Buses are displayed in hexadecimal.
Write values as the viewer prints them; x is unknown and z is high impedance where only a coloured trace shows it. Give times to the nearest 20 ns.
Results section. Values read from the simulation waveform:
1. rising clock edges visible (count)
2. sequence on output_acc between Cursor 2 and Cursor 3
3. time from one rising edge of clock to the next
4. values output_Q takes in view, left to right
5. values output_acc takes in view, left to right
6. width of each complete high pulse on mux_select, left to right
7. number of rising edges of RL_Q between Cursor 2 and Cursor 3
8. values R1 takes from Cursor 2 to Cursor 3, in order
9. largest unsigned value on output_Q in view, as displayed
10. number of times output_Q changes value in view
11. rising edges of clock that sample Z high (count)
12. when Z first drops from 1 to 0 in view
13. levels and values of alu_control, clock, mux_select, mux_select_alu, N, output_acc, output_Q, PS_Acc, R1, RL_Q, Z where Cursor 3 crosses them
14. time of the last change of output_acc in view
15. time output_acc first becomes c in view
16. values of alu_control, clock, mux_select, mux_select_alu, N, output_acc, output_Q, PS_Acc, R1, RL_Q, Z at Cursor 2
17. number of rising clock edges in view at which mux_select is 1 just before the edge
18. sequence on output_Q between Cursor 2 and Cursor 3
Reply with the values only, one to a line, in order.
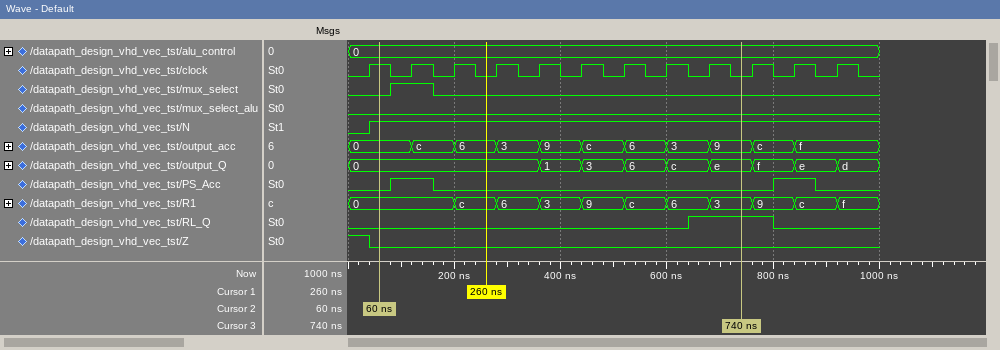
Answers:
12
0, c, 6, 3, 9, c, 6, 3, 9
80 ns
0, 1, 3, 6, c, e, f, e, d
0, c, 6, 3, 9, c, 6, 3, 9, c, f
80 ns
1
0, c, 6, 3, 9, c, 6, 3
f
8
1
40 ns
alu_control=0, clock=0, mux_select=0, mux_select_alu=0, N=1, output_acc=9, output_Q=e, PS_Acc=0, R1=3, RL_Q=1, Z=0
840 ns
120 ns
alu_control=0, clock=1, mux_select=0, mux_select_alu=0, N=1, output_acc=0, output_Q=0, PS_Acc=0, R1=0, RL_Q=0, Z=0
1
0, 1, 3, 6, c, e
